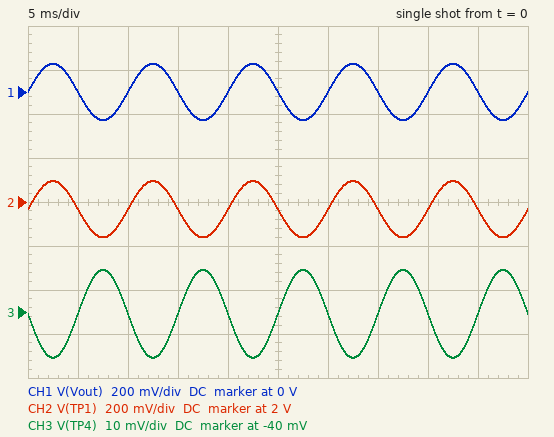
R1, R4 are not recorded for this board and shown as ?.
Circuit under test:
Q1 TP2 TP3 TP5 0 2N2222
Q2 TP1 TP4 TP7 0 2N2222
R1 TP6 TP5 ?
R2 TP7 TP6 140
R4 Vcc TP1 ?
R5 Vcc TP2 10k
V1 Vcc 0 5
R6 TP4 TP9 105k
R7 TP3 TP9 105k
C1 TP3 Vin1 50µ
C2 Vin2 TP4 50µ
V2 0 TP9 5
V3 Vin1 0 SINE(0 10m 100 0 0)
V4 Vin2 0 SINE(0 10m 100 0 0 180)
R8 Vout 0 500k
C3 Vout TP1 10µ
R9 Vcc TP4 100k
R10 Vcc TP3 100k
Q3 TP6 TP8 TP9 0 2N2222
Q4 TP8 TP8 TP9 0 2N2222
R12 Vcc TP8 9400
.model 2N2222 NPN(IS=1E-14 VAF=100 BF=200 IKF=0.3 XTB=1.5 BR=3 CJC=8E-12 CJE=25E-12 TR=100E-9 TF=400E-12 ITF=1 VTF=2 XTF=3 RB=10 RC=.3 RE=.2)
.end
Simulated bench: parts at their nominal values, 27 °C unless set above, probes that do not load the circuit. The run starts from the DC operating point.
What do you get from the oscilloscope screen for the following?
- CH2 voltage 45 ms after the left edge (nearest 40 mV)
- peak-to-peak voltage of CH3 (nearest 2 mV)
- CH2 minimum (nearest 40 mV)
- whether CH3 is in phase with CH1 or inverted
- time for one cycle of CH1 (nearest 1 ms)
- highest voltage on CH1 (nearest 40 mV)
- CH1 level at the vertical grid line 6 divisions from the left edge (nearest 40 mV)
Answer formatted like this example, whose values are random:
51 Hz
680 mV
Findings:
1.96 V
20 mV
1.84 V
inverted
10 ms
120 mV
0 V
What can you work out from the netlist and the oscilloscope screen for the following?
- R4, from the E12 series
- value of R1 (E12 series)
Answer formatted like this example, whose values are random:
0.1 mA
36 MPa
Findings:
4.7 kΩ
470 Ω
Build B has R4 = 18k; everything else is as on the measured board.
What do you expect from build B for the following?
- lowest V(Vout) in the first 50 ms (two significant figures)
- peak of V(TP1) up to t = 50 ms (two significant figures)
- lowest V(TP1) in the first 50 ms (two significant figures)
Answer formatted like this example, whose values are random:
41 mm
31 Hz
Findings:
-12 mV
-1.4 V
-1.5 V
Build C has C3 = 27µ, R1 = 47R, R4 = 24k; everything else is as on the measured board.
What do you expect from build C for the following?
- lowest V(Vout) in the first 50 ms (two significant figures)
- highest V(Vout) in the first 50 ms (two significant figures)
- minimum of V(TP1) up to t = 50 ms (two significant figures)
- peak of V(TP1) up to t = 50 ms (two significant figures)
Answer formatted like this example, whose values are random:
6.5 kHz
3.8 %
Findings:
-17 mV
260 mV
-1.8 V
-1.5 V
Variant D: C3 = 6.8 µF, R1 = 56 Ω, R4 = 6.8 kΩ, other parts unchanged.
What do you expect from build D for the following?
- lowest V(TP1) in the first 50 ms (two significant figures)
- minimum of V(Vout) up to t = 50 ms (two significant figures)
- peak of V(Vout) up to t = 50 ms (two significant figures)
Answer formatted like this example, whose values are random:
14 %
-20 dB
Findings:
1.2 V
-590 mV
320 mV
